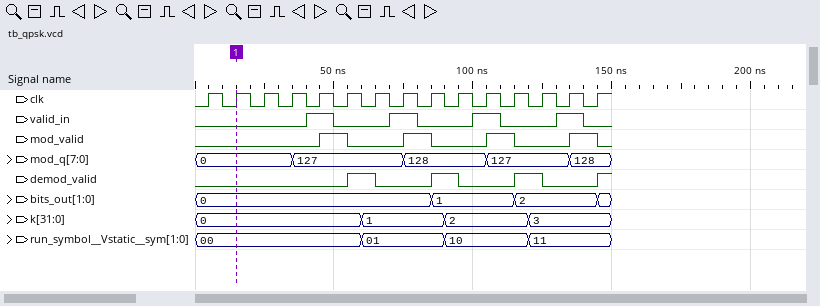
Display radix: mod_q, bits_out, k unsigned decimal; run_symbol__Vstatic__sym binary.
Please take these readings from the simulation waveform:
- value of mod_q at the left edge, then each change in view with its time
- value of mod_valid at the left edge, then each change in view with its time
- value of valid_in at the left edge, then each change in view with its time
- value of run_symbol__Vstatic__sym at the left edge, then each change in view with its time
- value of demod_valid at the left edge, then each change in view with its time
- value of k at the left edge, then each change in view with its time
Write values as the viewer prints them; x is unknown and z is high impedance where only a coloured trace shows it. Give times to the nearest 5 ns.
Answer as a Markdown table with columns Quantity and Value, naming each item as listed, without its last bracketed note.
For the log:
| Quantity | Value |
|---|---|
| value of mod_q at the left edge, then each change in view with its time | 0, 127 at 35 ns, 128 at 75 ns, 127 at 105 ns, 128 at 135 ns |
| value of mod_valid at the left edge, then each change in view with its time | 0, 1 at 45 ns, 0 at 55 ns, 1 at 75 ns, 0 at 85 ns, 1 at 105 ns, 0 at 115 ns, 1 at 135 ns, 0 at 145 ns |
| value of valid_in at the left edge, then each change in view with its time | 0, 1 at 40 ns, 0 at 50 ns, 1 at 70 ns, 0 at 80 ns, 1 at 100 ns, 0 at 110 ns, 1 at 130 ns, 0 at 140 ns |
| value of run_symbol__Vstatic__sym at the left edge, then each change in view with its time | 00, 01 at 60 ns, 10 at 90 ns, 11 at 120 ns |
| value of demod_valid at the left edge, then each change in view with its time | 0, 1 at 55 ns, 0 at 65 ns, 1 at 85 ns, 0 at 95 ns, 1 at 115 ns, 0 at 125 ns, 1 at 145 ns |
| value of k at the left edge, then each change in view with its time | 0, 1 at 60 ns, 2 at 90 ns, 3 at 120 ns |
